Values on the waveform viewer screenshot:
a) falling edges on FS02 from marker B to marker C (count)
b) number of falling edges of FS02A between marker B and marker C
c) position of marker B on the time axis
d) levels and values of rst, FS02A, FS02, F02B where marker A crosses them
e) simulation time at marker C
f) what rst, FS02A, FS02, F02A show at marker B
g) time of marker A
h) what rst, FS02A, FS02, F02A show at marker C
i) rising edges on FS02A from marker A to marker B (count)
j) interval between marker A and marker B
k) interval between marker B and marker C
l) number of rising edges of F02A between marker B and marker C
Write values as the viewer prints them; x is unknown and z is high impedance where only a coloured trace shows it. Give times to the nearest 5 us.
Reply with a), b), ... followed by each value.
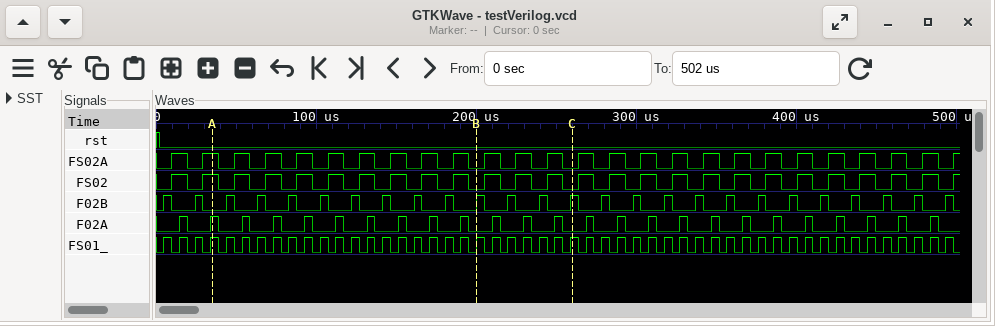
a) 3
b) 3
c) 200 us
d) rst=0, FS02A=1, FS02=1, F02B=0
e) 260 us
f) rst=0, FS02A=0, FS02=0, F02A=0
g) 35 us
h) rst=0, FS02A=0, FS02=0, F02A=0
i) 8
j) 165 us
k) 60 us
l) 3
